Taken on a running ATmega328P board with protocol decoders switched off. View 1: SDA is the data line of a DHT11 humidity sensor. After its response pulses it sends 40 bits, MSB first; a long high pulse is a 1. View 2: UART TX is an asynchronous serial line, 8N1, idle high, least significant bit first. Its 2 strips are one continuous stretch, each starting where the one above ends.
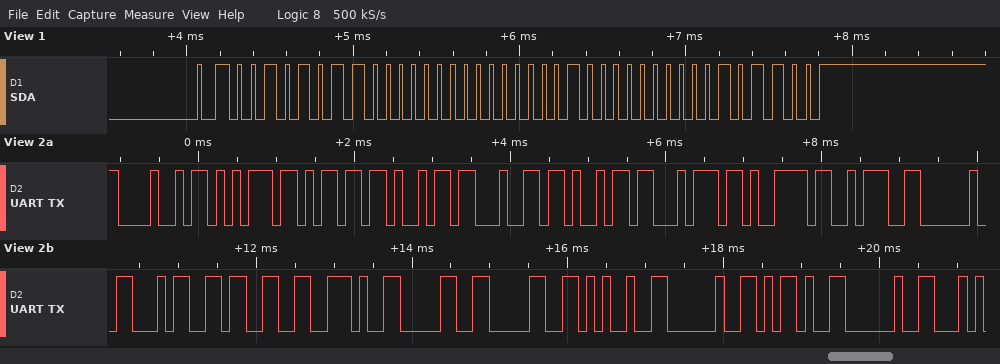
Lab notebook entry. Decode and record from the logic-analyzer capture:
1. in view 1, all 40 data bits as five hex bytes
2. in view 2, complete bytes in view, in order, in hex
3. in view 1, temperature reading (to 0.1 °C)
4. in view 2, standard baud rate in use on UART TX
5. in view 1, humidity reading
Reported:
2B 00 01 00 2C
0x48 0x75 0x6D 0x69 0x64 0x69 0x74 0x79 0x3A 0x20 0x34 0x33 0x2E 0x30 0x30 0x25 0x20 0x2D 0x20
1.0 °C
9600 baud
43 %
